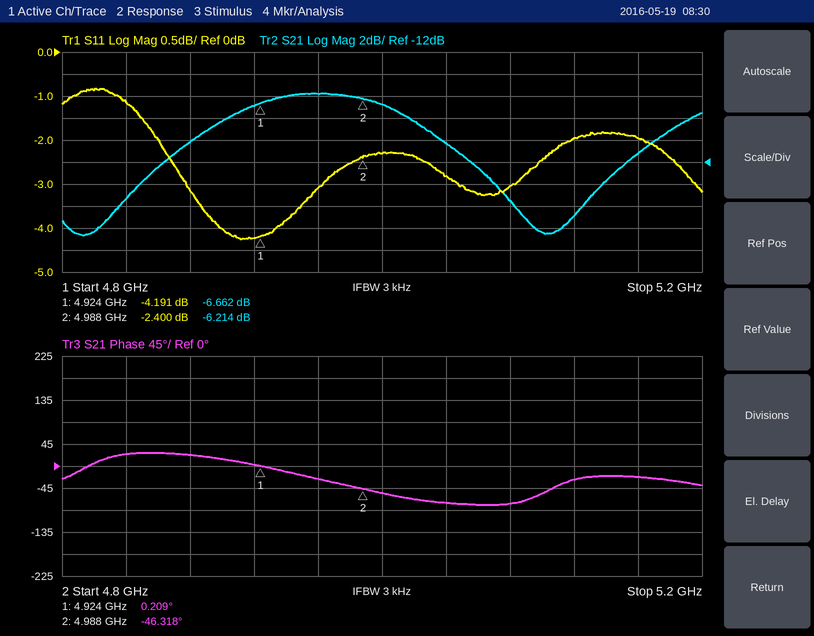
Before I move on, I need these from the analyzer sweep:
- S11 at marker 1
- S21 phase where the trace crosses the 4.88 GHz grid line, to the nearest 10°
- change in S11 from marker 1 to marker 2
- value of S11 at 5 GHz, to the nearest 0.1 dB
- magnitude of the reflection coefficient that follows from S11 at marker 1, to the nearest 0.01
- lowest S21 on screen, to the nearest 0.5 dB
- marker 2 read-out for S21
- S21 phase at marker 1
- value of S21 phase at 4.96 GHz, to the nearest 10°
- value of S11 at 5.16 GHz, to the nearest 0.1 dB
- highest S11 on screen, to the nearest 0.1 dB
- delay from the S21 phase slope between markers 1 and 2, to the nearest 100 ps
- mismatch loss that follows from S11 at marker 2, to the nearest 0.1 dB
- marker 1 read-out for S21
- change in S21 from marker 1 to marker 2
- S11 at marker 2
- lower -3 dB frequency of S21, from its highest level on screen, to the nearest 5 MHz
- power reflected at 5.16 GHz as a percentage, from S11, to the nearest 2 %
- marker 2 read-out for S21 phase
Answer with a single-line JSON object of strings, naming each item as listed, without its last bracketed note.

{"S11 at marker 1": "-4.191 dB", "S21 phase where the trace crosses the 4.88 GHz grid line, to the nearest 10°": "20°", "change in S11 from marker 1 to marker 2": "1.791 dB", "value of S11 at 5 GHz, to the nearest 0.1 dB": "-2.3 dB", "magnitude of the reflection coefficient that follows from S11 at marker 1, to the nearest 0.01": "0.62", "lowest S21 on screen, to the nearest 0.5 dB": "-18.5 dB", "marker 2 read-out for S21": "-6.214 dB", "S21 phase at marker 1": "0.209°", "value of S21 phase at 4.96 GHz, to the nearest 10°": "-30°", "value of S11 at 5.16 GHz, to the nearest 0.1 dB": "-2.0 dB", "highest S11 on screen, to the nearest 0.1 dB": "-0.8 dB", "delay from the S21 phase slope between markers 1 and 2, to the nearest 100 ps": "2.0 ns", "mismatch loss that follows from S11 at marker 2, to the nearest 0.1 dB": "3.7 dB", "marker 1 read-out for S21": "-6.662 dB", "change in S21 from marker 1 to marker 2": "0.448 dB", "S11 at marker 2": "-2.400 dB", "lower -3 dB frequency of S21, from its highest level on screen, to the nearest 5 MHz": "4.895 GHz", "power reflected at 5.16 GHz as a percentage, from S11, to the nearest 2 %": "64 %", "marker 2 read-out for S21 phase": "-46.318°"}
